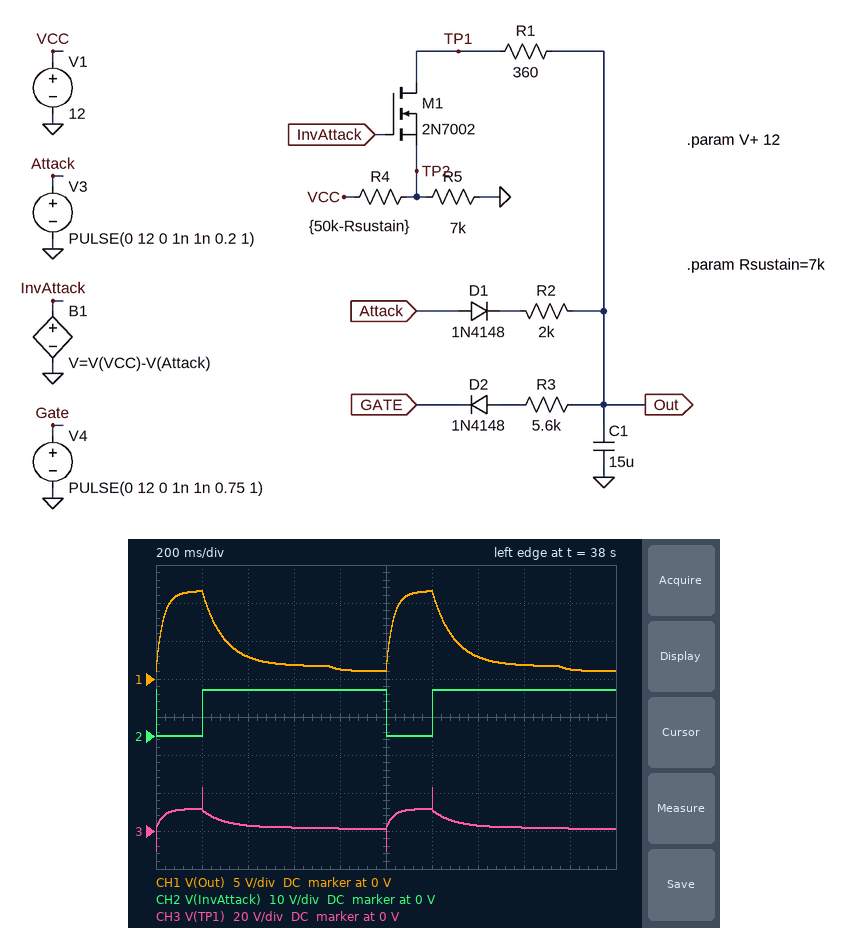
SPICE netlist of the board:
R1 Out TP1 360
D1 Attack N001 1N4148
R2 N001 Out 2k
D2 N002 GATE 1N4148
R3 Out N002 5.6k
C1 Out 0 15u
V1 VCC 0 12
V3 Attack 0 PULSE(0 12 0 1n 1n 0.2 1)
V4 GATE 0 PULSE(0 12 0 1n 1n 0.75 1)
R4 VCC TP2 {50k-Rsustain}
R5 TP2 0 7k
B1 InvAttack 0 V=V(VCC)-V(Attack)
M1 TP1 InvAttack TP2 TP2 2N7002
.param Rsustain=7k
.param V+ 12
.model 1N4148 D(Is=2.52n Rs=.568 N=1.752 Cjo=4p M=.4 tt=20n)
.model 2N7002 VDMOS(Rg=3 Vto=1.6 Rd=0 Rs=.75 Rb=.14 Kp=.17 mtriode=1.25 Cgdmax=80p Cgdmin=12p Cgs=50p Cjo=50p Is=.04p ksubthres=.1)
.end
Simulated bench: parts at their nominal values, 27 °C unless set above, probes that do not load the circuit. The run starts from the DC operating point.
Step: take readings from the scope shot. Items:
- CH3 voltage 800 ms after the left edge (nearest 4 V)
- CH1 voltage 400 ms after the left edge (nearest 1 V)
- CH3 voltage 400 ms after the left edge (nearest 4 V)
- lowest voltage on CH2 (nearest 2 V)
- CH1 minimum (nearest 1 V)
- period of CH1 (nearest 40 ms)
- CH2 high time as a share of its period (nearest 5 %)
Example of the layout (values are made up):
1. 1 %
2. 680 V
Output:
1. 0 V
2. 3 V
3. 4 V
4. 0 V
5. 1 V
6. 1.00 s
7. 80 %
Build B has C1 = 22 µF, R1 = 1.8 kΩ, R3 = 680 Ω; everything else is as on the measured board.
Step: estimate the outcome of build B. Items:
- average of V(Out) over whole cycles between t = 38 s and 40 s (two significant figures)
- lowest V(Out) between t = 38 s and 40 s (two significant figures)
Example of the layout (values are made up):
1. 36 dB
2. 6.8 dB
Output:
1. 4.5 V
2. 590 mV
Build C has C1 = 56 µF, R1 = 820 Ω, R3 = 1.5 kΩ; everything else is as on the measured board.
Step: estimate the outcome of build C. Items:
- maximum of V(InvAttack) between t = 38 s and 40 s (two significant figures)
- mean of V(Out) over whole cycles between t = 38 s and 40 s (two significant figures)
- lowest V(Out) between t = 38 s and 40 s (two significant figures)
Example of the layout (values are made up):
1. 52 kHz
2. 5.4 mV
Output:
1. 12 V
2. 4.9 V
3. 810 mV
